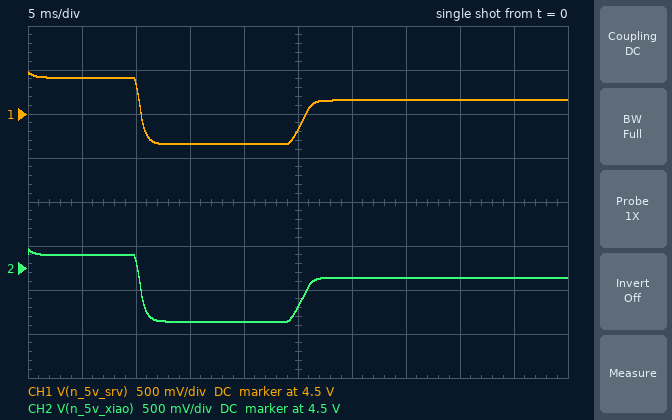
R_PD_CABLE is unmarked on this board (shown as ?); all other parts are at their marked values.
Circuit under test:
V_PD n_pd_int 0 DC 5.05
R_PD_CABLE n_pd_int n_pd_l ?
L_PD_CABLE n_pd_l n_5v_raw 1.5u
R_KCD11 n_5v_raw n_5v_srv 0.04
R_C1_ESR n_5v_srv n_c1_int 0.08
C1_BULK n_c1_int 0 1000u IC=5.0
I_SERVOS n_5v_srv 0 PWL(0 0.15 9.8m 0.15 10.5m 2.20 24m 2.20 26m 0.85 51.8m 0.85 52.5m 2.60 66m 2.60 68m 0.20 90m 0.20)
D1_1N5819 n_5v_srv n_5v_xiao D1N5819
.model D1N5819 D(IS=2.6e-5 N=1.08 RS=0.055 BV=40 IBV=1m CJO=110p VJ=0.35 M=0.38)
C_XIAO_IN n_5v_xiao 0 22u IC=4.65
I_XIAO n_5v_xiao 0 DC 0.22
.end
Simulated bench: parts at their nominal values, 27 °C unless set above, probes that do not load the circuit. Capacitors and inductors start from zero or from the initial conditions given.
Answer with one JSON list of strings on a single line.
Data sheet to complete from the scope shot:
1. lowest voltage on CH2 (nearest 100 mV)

["3.9 V"]
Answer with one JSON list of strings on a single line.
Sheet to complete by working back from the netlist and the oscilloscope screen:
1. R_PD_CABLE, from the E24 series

["0.33 Ω"]
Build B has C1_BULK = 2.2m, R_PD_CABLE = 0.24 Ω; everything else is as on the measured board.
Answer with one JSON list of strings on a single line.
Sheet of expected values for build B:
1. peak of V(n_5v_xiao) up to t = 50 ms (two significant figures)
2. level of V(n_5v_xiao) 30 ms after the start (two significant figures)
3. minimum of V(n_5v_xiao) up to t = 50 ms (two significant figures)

["4.7 V", "4.5 V", "4.1 V"]
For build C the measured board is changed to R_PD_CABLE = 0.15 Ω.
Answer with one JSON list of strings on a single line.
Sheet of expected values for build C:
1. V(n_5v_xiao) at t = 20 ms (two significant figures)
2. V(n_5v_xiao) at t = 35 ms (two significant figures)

["4.3 V", "4.6 V"]
